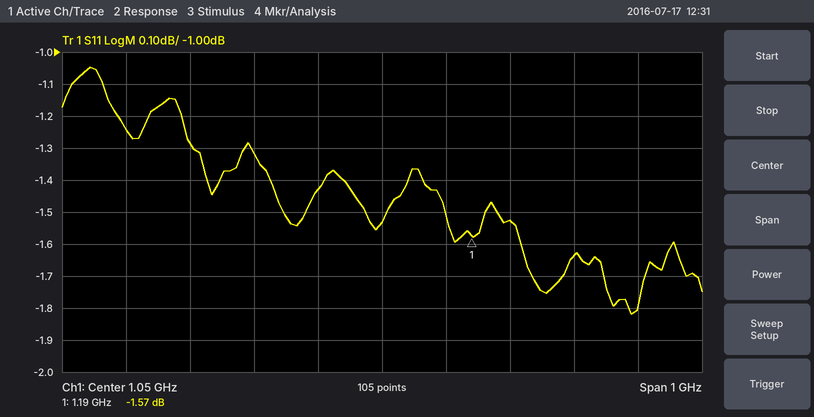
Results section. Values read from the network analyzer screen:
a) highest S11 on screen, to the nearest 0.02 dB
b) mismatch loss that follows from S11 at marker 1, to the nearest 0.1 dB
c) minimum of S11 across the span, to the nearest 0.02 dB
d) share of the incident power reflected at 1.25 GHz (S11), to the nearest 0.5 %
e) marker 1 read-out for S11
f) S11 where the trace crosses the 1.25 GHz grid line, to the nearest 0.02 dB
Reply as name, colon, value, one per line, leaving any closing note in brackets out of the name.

highest S11 on screen, to the nearest 0.02 dB: -1.04 dB
mismatch loss that follows from S11 at marker 1, to the nearest 0.1 dB: 5.2 dB
minimum of S11 across the span, to the nearest 0.02 dB: -1.82 dB
share of the incident power reflected at 1.25 GHz (S11), to the nearest 0.5 %: 70.5 %
marker 1 read-out for S11: -1.57 dB
S11 where the trace crosses the 1.25 GHz grid line, to the nearest 0.02 dB: -1.52 dB
